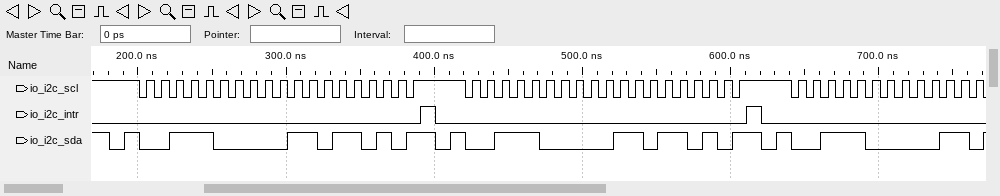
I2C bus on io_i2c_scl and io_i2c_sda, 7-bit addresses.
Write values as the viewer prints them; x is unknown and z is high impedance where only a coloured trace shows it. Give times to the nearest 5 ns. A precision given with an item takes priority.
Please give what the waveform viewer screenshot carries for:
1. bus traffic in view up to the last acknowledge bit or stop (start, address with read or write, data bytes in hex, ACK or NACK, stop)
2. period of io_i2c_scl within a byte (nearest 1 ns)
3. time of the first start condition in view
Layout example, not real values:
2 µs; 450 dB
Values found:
start, address 1C write ACK, 6D ACK, repeated start, address 1C write ACK, 6D ACK, repeated start, address 1C write ACK; 10 ns; 180 ns
